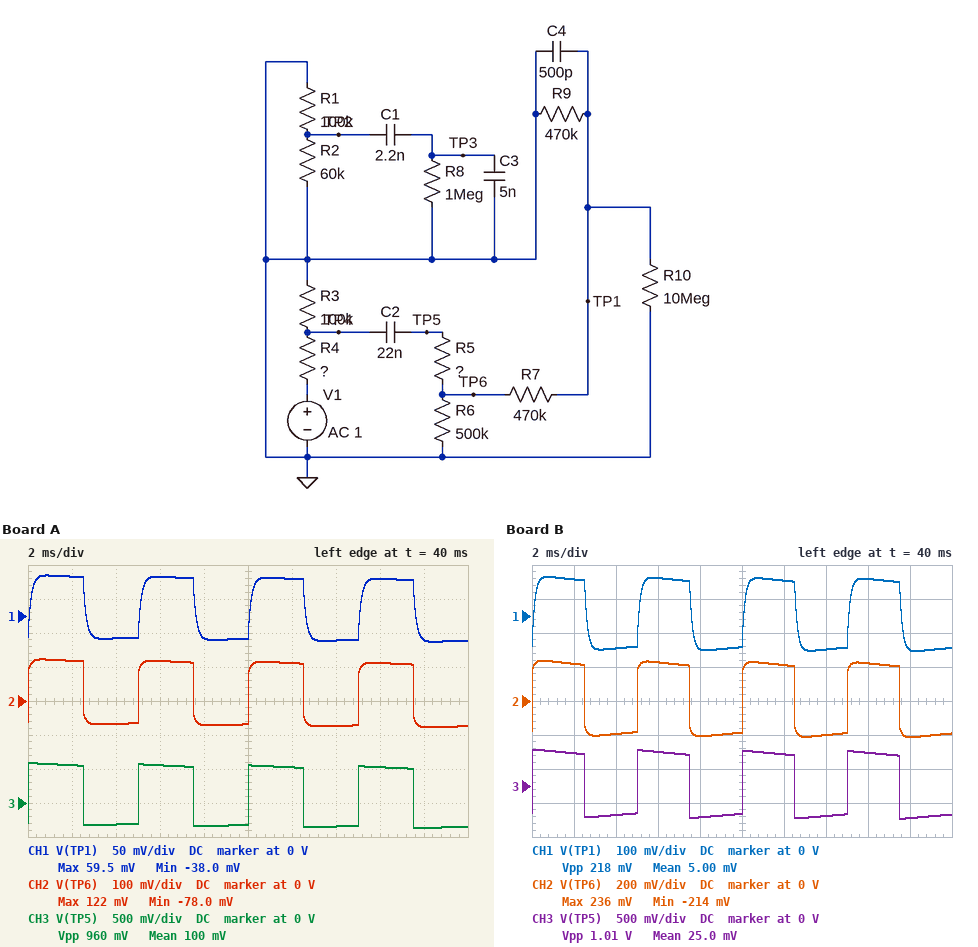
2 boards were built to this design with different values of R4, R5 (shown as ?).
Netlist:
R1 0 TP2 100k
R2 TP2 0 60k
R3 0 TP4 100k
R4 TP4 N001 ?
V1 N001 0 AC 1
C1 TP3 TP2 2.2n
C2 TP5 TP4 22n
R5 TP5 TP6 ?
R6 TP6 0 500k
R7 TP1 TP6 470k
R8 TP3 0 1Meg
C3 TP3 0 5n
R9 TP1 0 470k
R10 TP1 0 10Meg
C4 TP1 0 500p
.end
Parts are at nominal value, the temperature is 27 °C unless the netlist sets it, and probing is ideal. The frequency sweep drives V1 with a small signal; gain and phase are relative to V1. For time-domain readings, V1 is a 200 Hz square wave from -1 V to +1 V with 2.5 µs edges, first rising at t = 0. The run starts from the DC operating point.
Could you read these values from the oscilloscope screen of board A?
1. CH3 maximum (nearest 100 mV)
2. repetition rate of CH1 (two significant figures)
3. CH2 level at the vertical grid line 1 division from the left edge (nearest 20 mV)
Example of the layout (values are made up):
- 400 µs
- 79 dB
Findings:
- 600 mV
- 200 Hz
- 120 mV
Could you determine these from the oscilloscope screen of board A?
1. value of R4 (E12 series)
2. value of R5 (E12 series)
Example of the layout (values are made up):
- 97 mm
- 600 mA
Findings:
- 120 kΩ
- 1.2 MΩ
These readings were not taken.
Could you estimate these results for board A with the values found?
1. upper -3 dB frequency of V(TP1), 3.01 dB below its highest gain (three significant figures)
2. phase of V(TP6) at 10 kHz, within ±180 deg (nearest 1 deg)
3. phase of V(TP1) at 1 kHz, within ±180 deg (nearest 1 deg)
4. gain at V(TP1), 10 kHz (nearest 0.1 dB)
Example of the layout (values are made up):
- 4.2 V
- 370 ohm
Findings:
- 1.10 kHz
- -2 deg
- -42 deg
- -46.1 dB
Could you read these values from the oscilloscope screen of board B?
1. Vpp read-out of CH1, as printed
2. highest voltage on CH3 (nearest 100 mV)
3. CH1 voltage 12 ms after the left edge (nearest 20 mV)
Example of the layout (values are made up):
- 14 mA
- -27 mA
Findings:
- 218 mV
- 500 mV
- 100 mV
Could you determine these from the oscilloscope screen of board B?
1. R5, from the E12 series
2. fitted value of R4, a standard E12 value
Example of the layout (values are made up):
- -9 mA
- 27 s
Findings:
- 390 kΩ
- 100 kΩ
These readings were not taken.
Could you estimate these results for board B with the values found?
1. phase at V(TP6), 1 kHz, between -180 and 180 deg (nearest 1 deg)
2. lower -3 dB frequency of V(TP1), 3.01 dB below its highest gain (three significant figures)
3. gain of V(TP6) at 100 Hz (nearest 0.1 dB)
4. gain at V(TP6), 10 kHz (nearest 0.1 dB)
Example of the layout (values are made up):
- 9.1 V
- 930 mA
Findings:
- -4 deg
- 9.31 Hz
- -13.5 dB
- -15.0 dB
